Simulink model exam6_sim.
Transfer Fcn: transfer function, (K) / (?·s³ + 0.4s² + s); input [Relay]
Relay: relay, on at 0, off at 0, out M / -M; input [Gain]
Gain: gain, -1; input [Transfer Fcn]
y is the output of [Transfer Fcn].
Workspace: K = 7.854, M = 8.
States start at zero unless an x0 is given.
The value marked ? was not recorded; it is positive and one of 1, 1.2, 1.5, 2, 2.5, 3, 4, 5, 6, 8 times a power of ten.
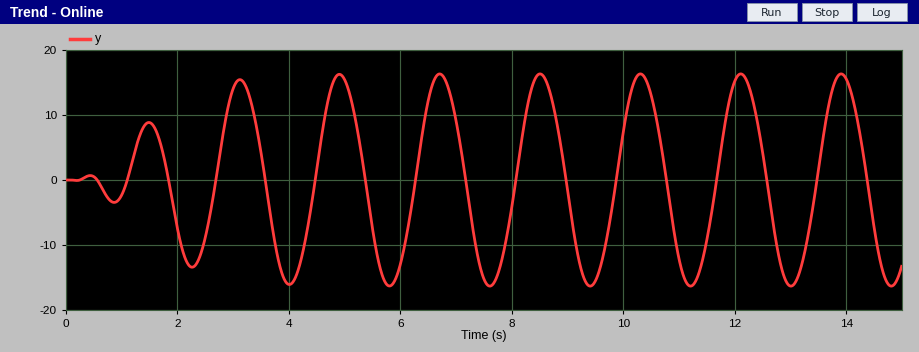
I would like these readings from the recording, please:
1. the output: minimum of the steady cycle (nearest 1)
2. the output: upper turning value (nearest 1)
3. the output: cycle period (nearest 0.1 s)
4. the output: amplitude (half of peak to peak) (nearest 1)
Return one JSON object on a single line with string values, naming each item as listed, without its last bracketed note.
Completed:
{"the output: minimum of the steady cycle": "-16", "the output: upper turning value": "16", "the output: cycle period": "1.8 s", "the output: amplitude (half of peak to peak)": "16"}
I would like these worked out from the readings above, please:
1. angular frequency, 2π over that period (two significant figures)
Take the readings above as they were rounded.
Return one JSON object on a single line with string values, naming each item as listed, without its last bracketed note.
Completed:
{"angular frequency, 2π over that period": "3.5 rad/s"}
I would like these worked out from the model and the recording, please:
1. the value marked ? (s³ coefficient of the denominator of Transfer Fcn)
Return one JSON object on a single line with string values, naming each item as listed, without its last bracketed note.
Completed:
{"the value marked ?": "0.08"}
